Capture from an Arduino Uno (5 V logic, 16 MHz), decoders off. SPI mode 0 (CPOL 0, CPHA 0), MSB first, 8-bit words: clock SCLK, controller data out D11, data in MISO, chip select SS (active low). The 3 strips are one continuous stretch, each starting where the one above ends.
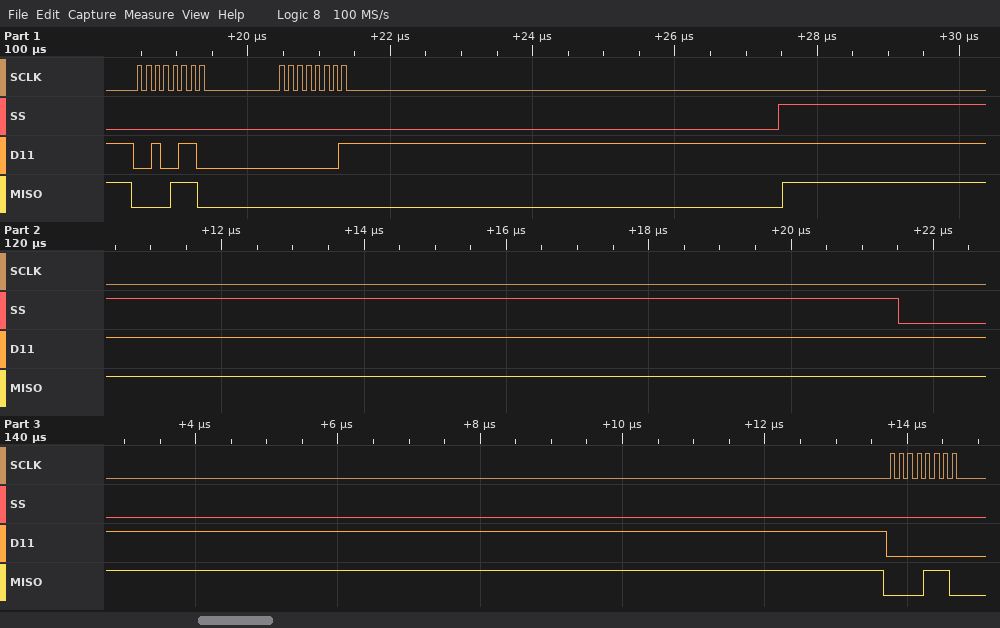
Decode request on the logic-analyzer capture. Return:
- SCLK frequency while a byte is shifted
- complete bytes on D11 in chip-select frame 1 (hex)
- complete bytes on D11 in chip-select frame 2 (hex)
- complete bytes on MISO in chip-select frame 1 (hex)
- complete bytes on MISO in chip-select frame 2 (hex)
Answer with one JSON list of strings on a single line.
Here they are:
["8 MHz", "26 01", "00", "0E 00", "0E"]
